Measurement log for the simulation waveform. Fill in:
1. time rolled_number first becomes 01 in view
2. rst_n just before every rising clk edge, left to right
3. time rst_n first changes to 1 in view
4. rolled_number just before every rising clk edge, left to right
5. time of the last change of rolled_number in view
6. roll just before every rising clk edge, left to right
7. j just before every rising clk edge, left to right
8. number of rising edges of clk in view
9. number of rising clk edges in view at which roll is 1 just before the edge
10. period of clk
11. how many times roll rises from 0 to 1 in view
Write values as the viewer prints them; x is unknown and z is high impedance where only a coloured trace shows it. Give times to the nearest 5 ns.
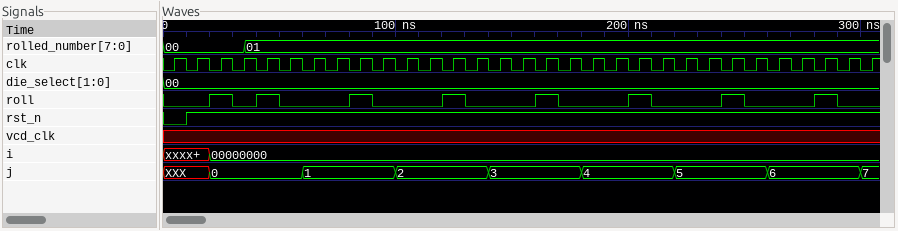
35 ns
0 1 1 1 1 1 1 1 1 1 1 1 1 1 1 1 1 1 1 1 1 1 1 1 1 1 1 1 1 1 1
10 ns
00, 00, 00, 00, 01, 01, 01, 01, 01, 01, 01, 01, 01, 01, 01, 01, 01, 01, 01, 01, 01, 01, 01, 01, 01, 01, 01, 01, 01, 01, 01
35 ns
0 0 1 0 1 0 0 0 1 0 0 0 1 0 0 0 1 0 0 0 1 0 0 0 1 0 0 0 1 0 0
XXX, XXX, 0, 0, 0, 0, 1, 1, 1, 1, 2, 2, 2, 2, 3, 3, 3, 3, 4, 4, 4, 4, 5, 5, 5, 5, 6, 6, 6, 6, 7
31
8
10 ns
8
